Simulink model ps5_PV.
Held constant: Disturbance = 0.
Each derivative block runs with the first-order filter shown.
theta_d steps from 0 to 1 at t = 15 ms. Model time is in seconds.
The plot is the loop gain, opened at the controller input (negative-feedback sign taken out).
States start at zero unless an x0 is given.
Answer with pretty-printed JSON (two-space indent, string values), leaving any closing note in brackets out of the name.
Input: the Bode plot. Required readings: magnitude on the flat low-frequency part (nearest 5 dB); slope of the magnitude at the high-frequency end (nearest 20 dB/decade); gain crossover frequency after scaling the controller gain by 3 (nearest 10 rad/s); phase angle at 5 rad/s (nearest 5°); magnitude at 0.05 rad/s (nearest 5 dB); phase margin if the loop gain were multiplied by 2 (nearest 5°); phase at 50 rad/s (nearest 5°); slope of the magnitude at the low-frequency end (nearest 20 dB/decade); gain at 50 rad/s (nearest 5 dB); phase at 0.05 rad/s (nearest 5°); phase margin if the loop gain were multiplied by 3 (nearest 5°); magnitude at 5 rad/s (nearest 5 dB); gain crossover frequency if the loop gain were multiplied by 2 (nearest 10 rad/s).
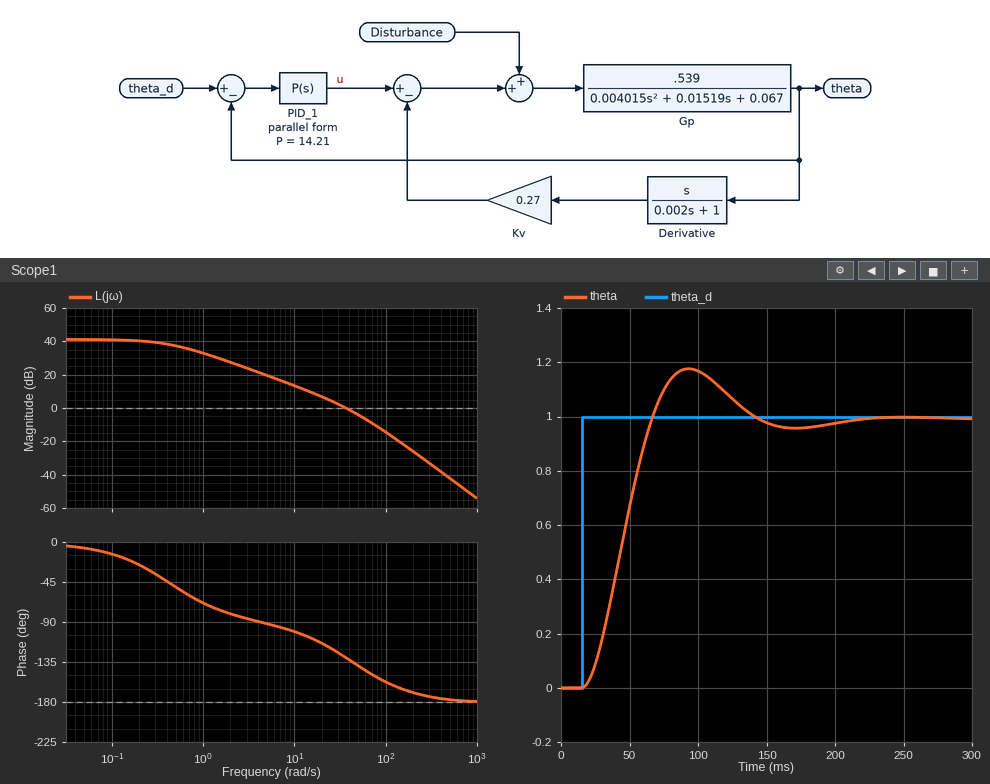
{
  "magnitude on the flat low-frequency part": "40 dB",
  "slope of the magnitude at the high-frequency end": "-40 dB/decade",
  "gain crossover frequency after scaling the controller gain by 3": "70 rad/s",
  "phase angle at 5 rad/s": "-90°",
  "magnitude at 0.05 rad/s": "40 dB",
  "phase margin if the loop gain were multiplied by 2": "35°",
  "phase at 50 rad/s": "-140°",
  "slope of the magnitude at the low-frequency end": "0 dB/decade",
  "gain at 50 rad/s": "-5 dB",
  "phase at 0.05 rad/s": "-5°",
  "phase margin if the loop gain were multiplied by 3": "30°",
  "magnitude at 5 rad/s": "20 dB",
  "gain crossover frequency if the loop gain were multiplied by 2": "60 rad/s"
}
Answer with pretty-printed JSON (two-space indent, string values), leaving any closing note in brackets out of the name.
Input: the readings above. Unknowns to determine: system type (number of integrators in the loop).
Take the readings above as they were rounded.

{
  "system type": "0"
}
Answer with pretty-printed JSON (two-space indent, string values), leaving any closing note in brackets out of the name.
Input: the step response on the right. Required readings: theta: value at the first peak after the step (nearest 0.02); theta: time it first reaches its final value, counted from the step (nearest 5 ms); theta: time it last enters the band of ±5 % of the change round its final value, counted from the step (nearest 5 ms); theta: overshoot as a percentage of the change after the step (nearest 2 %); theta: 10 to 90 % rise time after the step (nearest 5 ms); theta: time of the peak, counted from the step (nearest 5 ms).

{
  "theta: value at the first peak after the step": "1.18",
  "theta: time it first reaches its final value, counted from the step": "50 ms",
  "theta: time it last enters the band of ±5 % of the change round its final value, counted from the step": "115 ms",
  "theta: overshoot as a percentage of the change after the step": "18 %",
  "theta: 10 to 90 % rise time after the step": "35 ms",
  "theta: time of the peak, counted from the step": "80 ms"
}
